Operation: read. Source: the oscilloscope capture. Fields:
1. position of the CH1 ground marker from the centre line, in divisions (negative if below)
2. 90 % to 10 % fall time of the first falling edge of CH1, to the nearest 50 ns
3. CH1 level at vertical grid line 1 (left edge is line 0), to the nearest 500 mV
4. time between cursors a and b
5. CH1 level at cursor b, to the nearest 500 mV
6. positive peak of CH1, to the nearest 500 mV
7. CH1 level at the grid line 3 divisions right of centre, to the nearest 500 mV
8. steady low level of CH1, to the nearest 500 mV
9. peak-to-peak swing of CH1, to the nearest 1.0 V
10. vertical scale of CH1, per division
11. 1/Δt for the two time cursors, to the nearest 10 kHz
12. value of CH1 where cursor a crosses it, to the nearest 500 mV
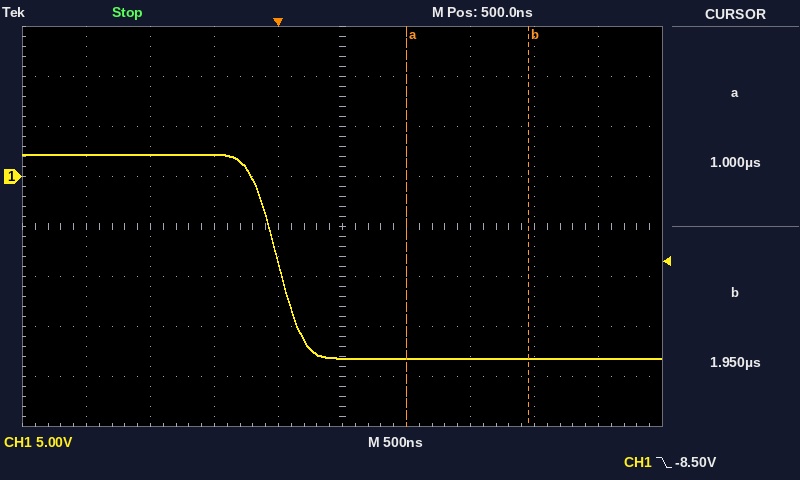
+1.0 div
400 ns
2.0 V
950 ns
-18.0 V
2.0 V
-18.0 V
-18.0 V
20.0 V
5 V
1.05 MHz
-18.0 V
